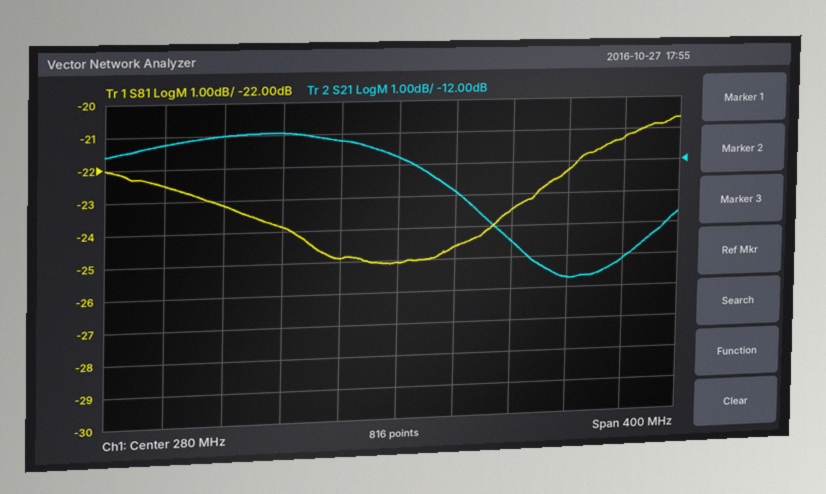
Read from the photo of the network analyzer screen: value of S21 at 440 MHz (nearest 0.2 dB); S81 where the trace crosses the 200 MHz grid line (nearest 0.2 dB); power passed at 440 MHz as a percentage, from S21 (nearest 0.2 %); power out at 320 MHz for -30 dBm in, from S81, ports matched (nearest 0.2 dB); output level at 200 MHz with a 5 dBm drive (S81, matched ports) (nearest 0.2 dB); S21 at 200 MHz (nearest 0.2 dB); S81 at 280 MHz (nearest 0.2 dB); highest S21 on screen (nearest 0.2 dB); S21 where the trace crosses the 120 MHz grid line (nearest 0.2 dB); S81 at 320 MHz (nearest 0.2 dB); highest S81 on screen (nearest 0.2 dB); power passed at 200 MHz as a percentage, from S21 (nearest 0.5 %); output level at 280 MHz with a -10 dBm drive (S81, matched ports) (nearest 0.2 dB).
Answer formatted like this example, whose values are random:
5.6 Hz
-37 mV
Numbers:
-15.2 dB
-23.8 dB
3.0 %
-54.6 dBm
-18.8 dBm
-11.0 dB
-25.0 dB
-11.0 dB
-11.2 dB
-24.6 dB
-20.6 dB
8.0 %
-35.0 dBm
